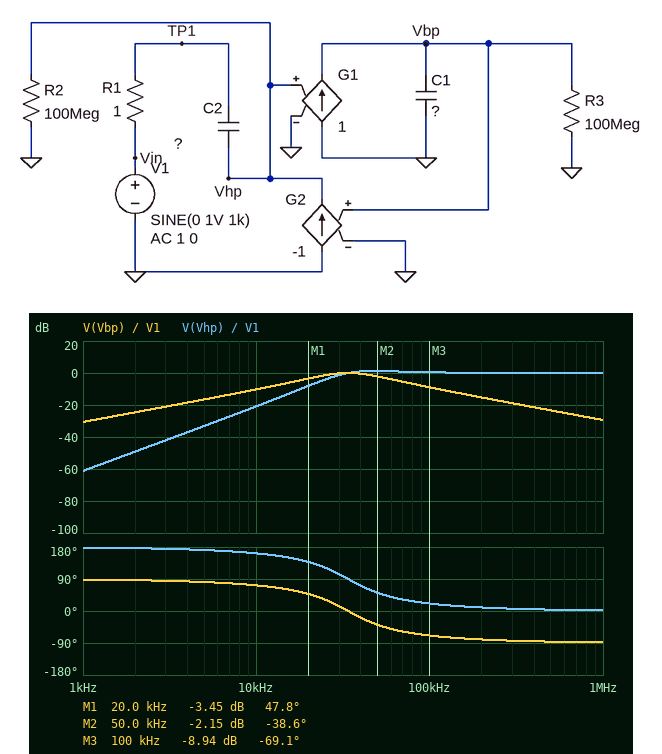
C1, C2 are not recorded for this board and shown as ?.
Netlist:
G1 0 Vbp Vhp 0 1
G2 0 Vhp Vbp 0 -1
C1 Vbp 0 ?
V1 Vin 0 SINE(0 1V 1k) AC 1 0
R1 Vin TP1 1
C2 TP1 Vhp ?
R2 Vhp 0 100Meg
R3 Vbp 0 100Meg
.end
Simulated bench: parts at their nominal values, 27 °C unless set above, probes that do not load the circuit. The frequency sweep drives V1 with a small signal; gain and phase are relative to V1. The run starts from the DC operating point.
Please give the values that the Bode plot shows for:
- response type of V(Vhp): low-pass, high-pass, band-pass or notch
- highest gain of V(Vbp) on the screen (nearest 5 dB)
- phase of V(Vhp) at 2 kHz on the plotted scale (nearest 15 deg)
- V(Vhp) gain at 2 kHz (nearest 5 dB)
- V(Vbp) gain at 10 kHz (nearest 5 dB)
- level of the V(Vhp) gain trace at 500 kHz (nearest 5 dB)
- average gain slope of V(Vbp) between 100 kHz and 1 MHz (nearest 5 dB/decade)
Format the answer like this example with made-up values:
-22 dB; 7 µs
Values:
high-pass; 0 dB; 180 deg; -50 dB; -10 dB; 0 dB; -20 dB/decade
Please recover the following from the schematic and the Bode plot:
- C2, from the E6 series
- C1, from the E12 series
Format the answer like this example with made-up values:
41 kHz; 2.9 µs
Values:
4.7 µF; 4.7 µF
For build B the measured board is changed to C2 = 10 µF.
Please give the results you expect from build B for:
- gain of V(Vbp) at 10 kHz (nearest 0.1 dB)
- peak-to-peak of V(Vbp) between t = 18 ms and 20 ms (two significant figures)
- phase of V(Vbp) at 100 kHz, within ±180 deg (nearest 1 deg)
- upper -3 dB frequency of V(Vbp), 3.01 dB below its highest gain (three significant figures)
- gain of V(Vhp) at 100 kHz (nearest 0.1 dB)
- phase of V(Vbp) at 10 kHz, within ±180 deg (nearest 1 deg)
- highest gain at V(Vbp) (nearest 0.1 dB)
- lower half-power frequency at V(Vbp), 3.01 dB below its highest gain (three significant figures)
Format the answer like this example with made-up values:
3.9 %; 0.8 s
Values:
-4.3 dB; 130 mV; -70 deg; 45.7 kHz; 0 dB; 52 deg; 0 dB; 11.8 kHz
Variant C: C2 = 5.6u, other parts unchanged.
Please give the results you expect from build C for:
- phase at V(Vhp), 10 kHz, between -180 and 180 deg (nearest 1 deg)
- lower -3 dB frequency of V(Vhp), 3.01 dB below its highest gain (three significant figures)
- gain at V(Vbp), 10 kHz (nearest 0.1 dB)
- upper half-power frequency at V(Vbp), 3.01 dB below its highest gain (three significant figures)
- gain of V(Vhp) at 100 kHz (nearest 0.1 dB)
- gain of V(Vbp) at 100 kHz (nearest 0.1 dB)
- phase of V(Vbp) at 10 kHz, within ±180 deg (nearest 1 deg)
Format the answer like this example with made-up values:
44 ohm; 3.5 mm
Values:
159 deg; 27.0 kHz; -8.7 dB; 52.3 kHz; 0.3 dB; -9.1 dB; 69 deg
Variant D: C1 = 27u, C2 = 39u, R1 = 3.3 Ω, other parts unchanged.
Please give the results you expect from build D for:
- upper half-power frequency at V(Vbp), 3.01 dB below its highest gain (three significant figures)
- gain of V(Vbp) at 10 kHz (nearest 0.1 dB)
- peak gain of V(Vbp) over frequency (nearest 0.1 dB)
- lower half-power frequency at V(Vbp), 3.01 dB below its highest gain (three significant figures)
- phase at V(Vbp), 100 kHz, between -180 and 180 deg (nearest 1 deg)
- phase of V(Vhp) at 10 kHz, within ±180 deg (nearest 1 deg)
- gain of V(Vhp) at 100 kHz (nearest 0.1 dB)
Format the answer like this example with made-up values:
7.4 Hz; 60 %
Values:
20.6 kHz; -11.0 dB; -10.4 dB; 1.17 kHz; -79 deg; 69 deg; -0.1 dB
